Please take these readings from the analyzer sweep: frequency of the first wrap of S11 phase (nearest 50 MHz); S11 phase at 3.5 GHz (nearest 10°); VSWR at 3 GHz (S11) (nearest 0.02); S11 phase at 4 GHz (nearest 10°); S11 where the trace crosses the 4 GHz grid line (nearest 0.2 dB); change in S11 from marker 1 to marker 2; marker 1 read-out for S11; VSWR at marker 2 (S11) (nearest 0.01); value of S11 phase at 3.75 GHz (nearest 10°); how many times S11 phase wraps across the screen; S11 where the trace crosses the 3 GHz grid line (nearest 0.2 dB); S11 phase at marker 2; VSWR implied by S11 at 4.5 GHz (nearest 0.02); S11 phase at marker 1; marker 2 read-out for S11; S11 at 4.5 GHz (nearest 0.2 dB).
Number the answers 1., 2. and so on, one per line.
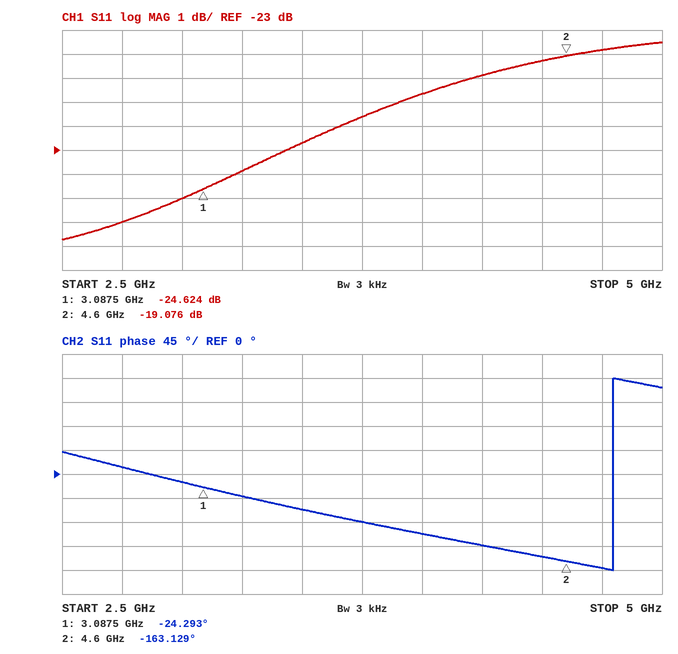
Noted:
1. 4.80 GHz
2. -70°
3. 1.12
4. -110°
5. -20.6 dB
6. 5.548 dB
7. -24.624 dB
8. 1.25
9. -90°
10. 1
11. -25.0 dB
12. -163.129°
13. 1.24
14. -24.293°
15. -19.076 dB
16. -19.2 dB
